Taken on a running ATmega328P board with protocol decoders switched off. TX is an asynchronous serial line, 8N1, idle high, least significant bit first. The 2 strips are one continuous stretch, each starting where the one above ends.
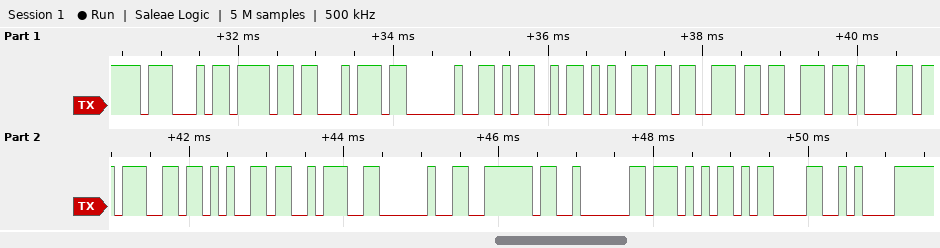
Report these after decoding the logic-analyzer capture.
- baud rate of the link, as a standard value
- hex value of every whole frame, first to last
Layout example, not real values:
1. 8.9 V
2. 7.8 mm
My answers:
1. 9600 baud
2. 0x47 0x6F 0x74 0x20 0x4D 0x65 0x73 0x73 0x61 0x67 0x65 0x3A 0x20 0x7E 0x02 0x57 0x0D 0x0A
